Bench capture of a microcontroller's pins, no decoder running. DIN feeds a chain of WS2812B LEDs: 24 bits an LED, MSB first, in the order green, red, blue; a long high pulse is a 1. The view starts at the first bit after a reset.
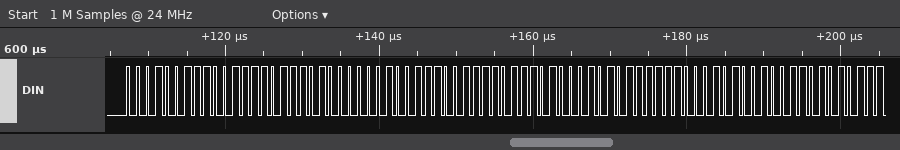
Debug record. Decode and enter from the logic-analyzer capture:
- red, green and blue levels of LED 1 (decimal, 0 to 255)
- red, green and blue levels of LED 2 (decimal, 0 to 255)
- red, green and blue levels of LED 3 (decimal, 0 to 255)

158, 19, 232
158, 19, 232
197, 175, 38
